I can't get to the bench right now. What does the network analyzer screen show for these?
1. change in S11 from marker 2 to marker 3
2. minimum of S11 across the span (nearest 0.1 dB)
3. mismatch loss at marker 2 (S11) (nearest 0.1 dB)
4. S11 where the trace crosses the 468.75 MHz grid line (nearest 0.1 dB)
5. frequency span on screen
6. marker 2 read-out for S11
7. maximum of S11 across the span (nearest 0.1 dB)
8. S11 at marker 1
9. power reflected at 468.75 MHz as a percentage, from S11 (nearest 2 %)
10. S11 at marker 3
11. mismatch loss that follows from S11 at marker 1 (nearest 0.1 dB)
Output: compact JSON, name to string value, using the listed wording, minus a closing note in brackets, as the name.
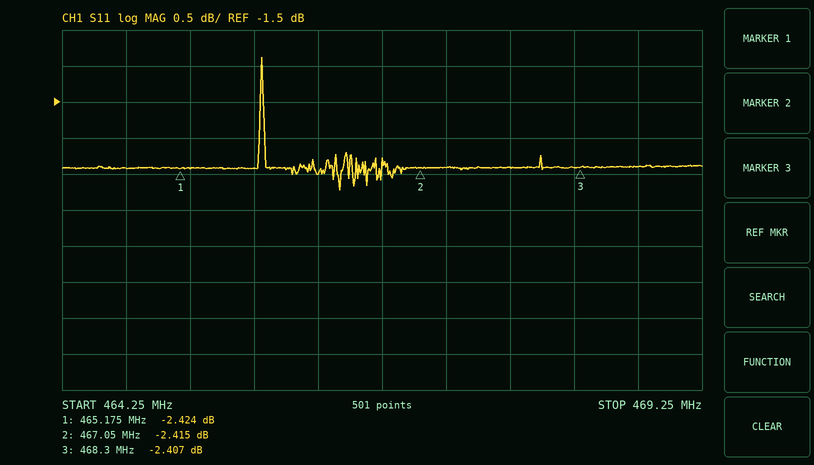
{"change in S11 from marker 2 to marker 3": "0.008 dB", "minimum of S11 across the span": "-2.7 dB", "mismatch loss at marker 2 (S11)": "3.7 dB", "S11 where the trace crosses the 468.75 MHz grid line": "-2.4 dB", "frequency span on screen": "5 MHz", "marker 2 read-out for S11": "-2.415 dB", "maximum of S11 across the span": "-0.9 dB", "S11 at marker 1": "-2.424 dB", "power reflected at 468.75 MHz as a percentage, from S11": "58 %", "S11 at marker 3": "-2.407 dB", "mismatch loss that follows from S11 at marker 1": "3.7 dB"}
